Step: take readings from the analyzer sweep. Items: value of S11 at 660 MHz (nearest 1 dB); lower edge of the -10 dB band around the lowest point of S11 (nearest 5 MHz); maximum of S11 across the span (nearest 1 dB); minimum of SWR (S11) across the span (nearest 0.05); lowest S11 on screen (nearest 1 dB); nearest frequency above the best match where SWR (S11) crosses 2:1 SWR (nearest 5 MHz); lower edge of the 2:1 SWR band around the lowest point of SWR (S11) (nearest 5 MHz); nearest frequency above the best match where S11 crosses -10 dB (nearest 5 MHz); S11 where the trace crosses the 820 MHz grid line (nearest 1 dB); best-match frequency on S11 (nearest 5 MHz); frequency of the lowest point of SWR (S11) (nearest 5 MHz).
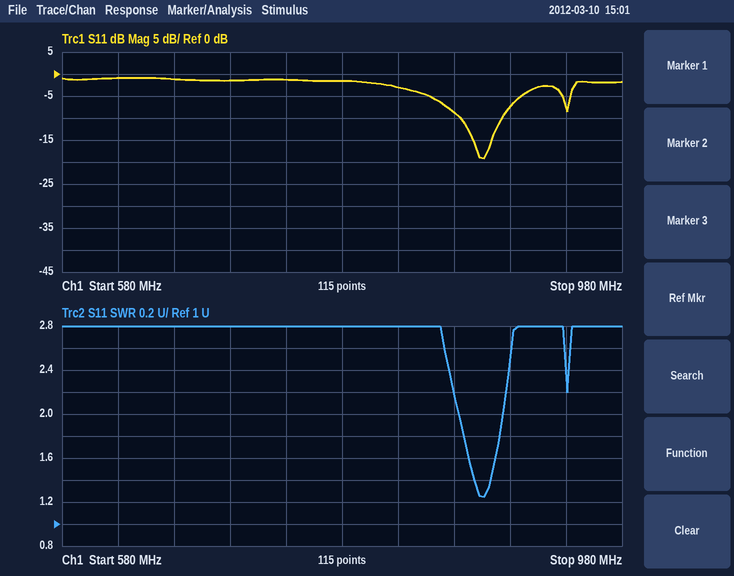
-1 dB
865 MHz
-1 dB
1.25
-19 dB
895 MHz
865 MHz
895 MHz
-3 dB
880 MHz
880 MHz
